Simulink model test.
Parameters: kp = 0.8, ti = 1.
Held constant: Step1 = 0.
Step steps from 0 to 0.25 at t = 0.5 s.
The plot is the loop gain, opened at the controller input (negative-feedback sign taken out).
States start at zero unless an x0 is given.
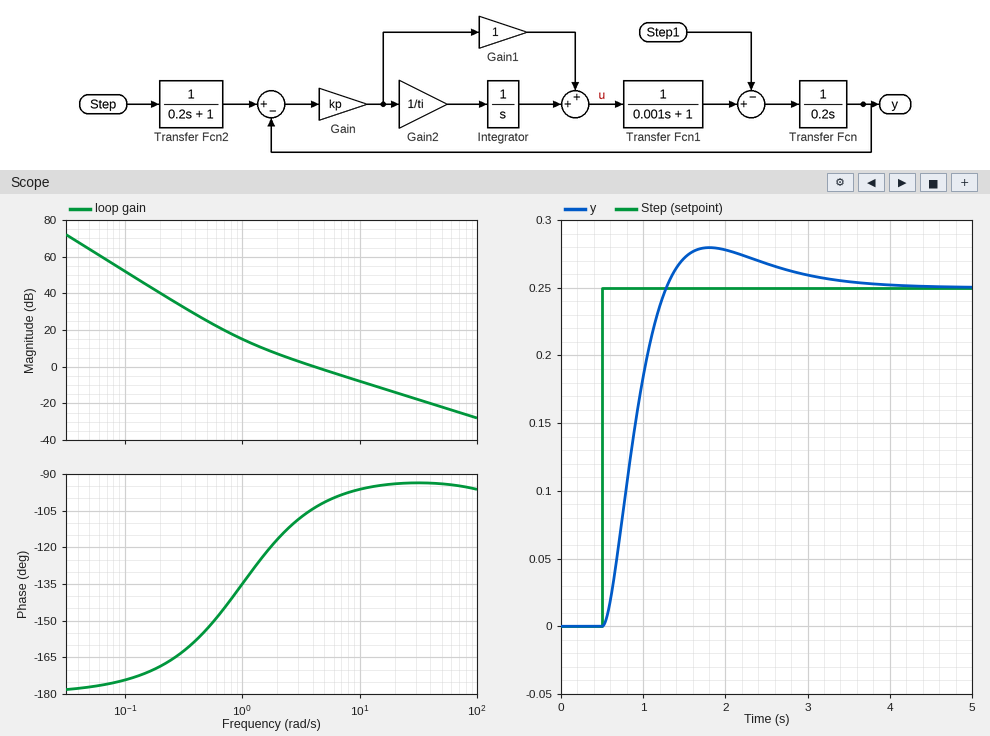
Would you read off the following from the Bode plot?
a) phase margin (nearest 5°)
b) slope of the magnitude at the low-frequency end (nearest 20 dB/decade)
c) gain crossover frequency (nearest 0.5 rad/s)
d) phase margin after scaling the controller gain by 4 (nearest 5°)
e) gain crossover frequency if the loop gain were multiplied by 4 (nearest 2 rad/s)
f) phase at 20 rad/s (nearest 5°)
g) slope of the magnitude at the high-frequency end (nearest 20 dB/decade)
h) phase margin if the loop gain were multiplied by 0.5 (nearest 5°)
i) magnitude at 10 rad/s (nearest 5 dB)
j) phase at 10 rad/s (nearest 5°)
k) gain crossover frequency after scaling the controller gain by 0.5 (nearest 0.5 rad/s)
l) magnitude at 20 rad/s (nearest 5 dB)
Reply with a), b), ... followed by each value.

a) 75°
b) -40 dB/decade
c) 4.0 rad/s
d) 85°
e) 16 rad/s
f) -95°
g) -20 dB/decade
h) 65°
i) -10 dB
j) -95°
k) 2.0 rad/s
l) -15 dB
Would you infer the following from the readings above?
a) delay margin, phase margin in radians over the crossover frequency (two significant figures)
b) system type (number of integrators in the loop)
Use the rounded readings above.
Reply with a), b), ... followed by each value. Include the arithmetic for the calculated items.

a) 75 × π / 180 / 4 = 0.33 s
b) 2
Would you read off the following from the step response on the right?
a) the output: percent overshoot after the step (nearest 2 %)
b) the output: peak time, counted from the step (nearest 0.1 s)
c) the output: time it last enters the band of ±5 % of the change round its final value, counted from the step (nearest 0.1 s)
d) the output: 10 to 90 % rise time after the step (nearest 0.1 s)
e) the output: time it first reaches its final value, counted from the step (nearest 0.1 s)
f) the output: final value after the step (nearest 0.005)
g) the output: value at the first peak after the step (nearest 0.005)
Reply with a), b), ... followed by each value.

a) 12 %
b) 1.3 s
c) 2.3 s
d) 0.5 s
e) 0.8 s
f) 0.250
g) 0.280
